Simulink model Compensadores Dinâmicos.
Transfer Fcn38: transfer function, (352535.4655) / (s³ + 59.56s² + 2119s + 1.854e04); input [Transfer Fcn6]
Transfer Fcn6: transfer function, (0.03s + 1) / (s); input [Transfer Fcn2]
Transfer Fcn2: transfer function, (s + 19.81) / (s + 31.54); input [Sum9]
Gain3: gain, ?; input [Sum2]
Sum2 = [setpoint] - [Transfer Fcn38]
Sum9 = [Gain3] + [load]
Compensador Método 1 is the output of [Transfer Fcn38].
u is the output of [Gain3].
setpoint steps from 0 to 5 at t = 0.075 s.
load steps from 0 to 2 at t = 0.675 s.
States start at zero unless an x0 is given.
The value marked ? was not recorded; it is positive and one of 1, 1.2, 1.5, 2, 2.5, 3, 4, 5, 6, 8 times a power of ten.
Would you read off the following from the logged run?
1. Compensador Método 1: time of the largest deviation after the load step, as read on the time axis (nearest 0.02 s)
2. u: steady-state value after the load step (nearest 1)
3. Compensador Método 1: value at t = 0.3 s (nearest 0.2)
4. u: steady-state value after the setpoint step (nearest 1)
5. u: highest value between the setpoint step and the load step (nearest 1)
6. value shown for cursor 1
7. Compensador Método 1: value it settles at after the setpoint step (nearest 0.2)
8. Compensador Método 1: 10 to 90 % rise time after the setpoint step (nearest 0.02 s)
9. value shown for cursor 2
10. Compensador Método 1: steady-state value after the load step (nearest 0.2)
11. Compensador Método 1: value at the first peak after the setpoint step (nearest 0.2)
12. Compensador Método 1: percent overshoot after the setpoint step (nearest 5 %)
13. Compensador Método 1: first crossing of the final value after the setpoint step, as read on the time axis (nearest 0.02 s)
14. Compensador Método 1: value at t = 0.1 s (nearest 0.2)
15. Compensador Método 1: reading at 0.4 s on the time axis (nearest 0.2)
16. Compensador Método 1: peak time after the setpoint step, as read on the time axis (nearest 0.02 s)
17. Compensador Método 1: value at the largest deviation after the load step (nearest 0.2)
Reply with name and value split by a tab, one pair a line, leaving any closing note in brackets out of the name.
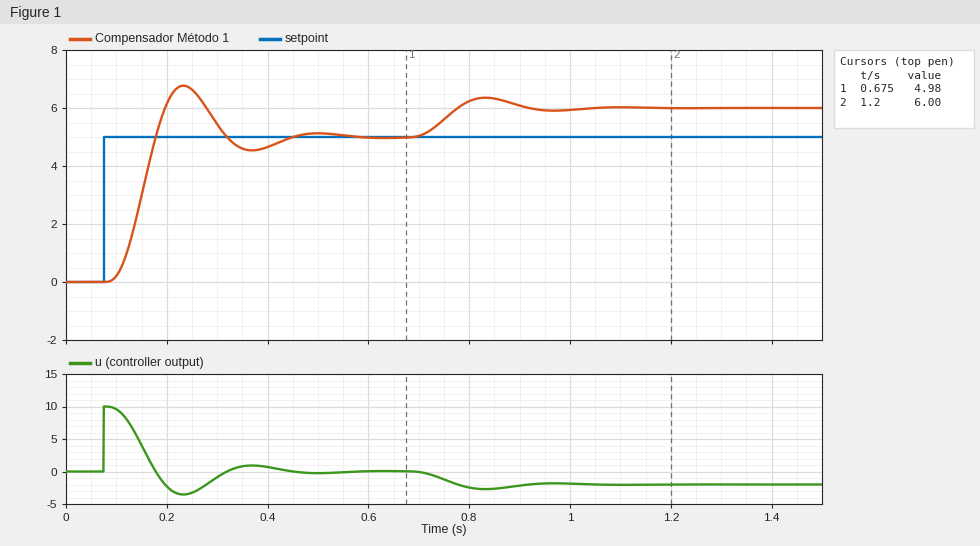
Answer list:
Compensador Método 1: time of the largest deviation after the load step, as read on the time axis	0.84 s
u: steady-state value after the load step	-2
Compensador Método 1: value at t = 0.3 s	5.4
u: steady-state value after the setpoint step	0
u: highest value between the setpoint step and the load step	10
value shown for cursor 1	4.98
Compensador Método 1: value it settles at after the setpoint step	5.0
Compensador Método 1: 10 to 90 % rise time after the setpoint step	0.06 s
value shown for cursor 2	6.00
Compensador Método 1: steady-state value after the load step	6.0
Compensador Método 1: value at the first peak after the setpoint step	6.8
Compensador Método 1: percent overshoot after the setpoint step	35 %
Compensador Método 1: first crossing of the final value after the setpoint step, as read on the time axis	0.18 s
Compensador Método 1: value at t = 0.1 s	0.2
Compensador Método 1: reading at 0.4 s on the time axis	4.6
Compensador Método 1: peak time after the setpoint step, as read on the time axis	0.24 s
Compensador Método 1: value at the largest deviation after the load step	6.4
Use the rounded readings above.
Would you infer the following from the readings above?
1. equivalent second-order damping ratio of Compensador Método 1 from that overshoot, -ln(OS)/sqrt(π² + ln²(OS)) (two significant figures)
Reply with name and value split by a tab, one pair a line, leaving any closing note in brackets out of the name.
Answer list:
equivalent second-order damping ratio of Compensador Método 1 from that overshoot, -ln(OS)/sqrt(π² + ln²(OS))	0.32
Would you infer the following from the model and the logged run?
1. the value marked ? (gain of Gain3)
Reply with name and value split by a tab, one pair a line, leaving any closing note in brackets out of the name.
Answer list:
the value marked ?	2
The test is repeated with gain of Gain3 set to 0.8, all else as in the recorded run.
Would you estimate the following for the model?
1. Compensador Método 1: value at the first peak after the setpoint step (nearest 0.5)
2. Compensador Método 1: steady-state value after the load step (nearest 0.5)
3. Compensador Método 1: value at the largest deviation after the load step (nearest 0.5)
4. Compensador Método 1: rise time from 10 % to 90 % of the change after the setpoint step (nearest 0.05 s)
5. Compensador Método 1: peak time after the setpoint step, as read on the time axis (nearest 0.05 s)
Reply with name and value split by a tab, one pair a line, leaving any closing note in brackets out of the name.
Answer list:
Compensador Método 1: value at the first peak after the setpoint step	5.5
Compensador Método 1: steady-state value after the load step	7.5
Compensador Método 1: value at the largest deviation after the load step	7.5
Compensador Método 1: rise time from 10 % to 90 % of the change after the setpoint step	0.15 s
Compensador Método 1: peak time after the setpoint step, as read on the time axis	0.40 s
